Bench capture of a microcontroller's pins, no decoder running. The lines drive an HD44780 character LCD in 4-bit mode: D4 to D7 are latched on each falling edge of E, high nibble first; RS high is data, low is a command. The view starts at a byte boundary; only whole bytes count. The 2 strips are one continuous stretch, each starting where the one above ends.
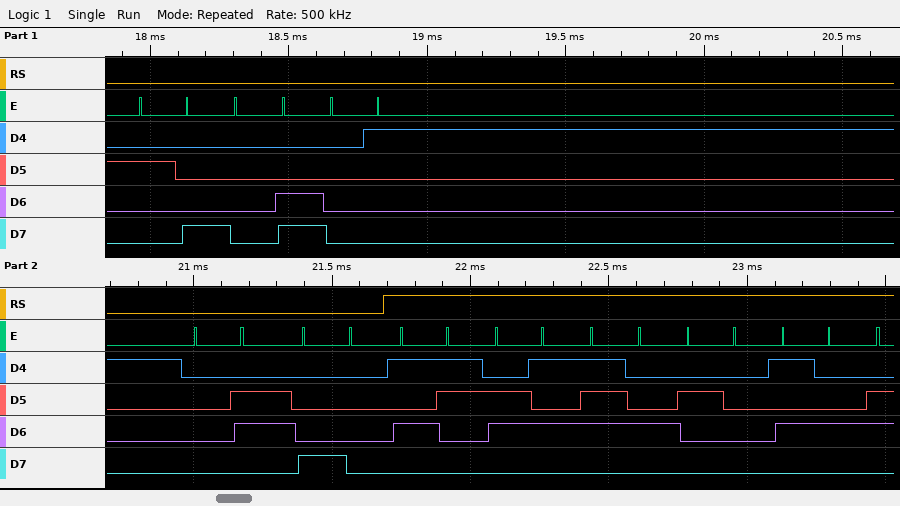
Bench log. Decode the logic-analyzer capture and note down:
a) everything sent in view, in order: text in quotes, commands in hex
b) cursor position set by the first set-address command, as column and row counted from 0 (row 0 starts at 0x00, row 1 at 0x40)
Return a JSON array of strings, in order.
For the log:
["0x28 0x0C 0x01 0x06 0x80 \"Set T\"", "column 0, row 0"]
